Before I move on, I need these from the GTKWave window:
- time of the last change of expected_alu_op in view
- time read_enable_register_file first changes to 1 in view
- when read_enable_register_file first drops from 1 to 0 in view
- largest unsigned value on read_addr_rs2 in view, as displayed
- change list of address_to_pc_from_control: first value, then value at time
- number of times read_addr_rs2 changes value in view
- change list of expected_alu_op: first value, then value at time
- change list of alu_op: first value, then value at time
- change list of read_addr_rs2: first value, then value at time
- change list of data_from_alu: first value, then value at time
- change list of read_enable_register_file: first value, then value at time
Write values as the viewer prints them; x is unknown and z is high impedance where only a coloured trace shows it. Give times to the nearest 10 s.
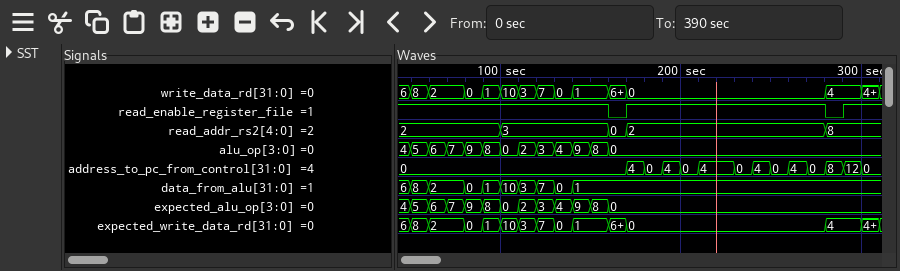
160 s
170 s
160 s
8
0, 4 at 170 s, 0 at 180 s, 4 at 190 s, 0 at 200 s, 4 at 210 s, 0 at 230 s, 4 at 240 s, 0 at 250 s, 4 at 260 s, 0 at 270 s, 8 at 280 s, 12 at 290 s, 0 at 300 s
4
4, 5 at 50 s, 6 at 60 s, 7 at 70 s, 9 at 80 s, 8 at 90 s, 0 at 100 s, 2 at 110 s, 3 at 120 s, 4 at 130 s, 9 at 140 s, 8 at 150 s, 0 at 160 s
4, 5 at 50 s, 6 at 60 s, 7 at 70 s, 9 at 80 s, 8 at 90 s, 0 at 100 s, 2 at 110 s, 3 at 120 s, 4 at 130 s, 9 at 140 s, 8 at 150 s, 0 at 160 s
2, 3 at 100 s, 0 at 160 s, 2 at 170 s, 8 at 280 s
6, 8 at 50 s, 2 at 60 s, 0 at 80 s, 1 at 90 s, 10 at 100 s, 3 at 110 s, 7 at 120 s, 0 at 130 s, 1 at 140 s
1, 0 at 160 s, 1 at 170 s, 0 at 280 s, 1 at 290 s
